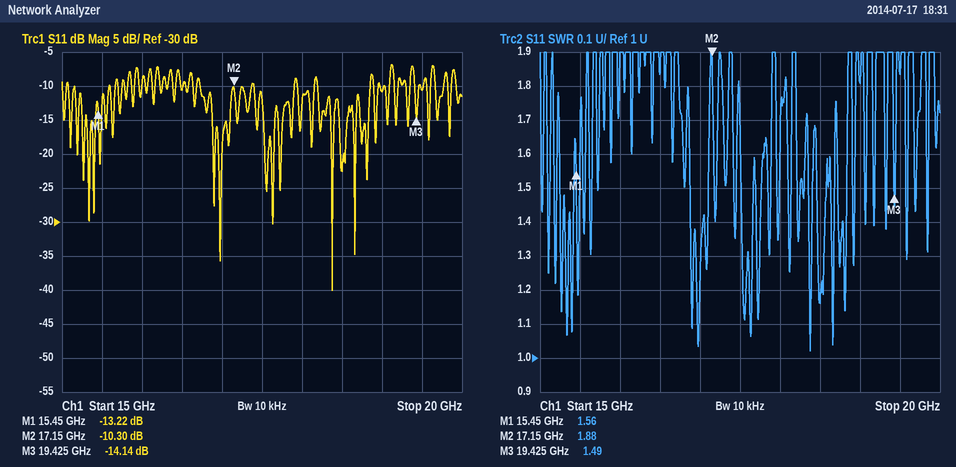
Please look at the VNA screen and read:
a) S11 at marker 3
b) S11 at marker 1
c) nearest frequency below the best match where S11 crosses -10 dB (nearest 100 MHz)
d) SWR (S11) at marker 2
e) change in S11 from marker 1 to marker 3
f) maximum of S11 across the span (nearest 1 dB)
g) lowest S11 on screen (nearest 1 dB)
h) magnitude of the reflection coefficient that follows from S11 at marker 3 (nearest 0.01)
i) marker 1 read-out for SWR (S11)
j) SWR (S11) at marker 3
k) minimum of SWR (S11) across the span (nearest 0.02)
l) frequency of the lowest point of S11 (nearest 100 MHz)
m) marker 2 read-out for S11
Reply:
-14.14 dB
-13.22 dB
18.2 GHz
1.88
-0.92 dB
-7 dB
-40 dB
0.20
1.56
1.49
1.02
18.4 GHz
-10.30 dB
